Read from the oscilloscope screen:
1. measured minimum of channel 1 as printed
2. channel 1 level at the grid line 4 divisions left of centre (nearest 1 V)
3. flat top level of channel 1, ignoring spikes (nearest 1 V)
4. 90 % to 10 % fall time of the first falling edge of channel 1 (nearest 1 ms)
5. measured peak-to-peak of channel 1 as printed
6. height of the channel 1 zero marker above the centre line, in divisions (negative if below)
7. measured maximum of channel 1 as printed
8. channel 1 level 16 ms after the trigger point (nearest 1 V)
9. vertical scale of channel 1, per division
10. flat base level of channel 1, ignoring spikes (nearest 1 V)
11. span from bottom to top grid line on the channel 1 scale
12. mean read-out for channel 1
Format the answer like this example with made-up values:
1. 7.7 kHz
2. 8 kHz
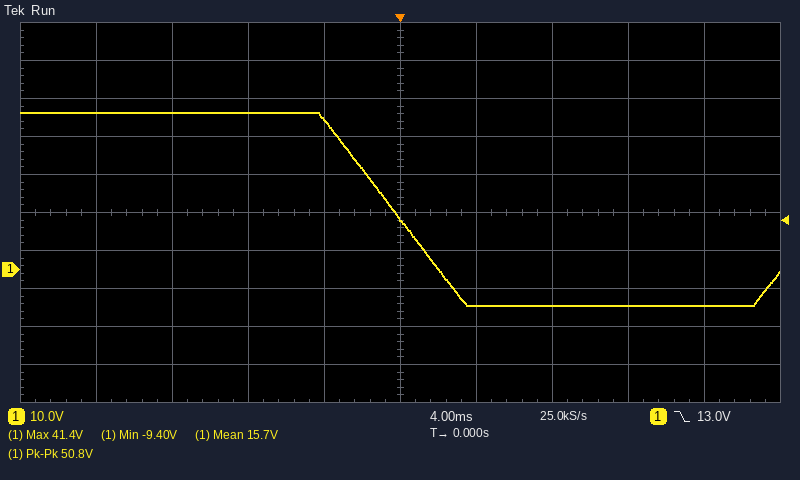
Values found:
1. -9.40 V
2. 41 V
3. 41 V
4. 6 ms
5. 50.8 V
6. -1.5 div
7. 41.4 V
8. -9 V
9. 10 V
10. -9 V
11. 100 V
12. 15.7 V
